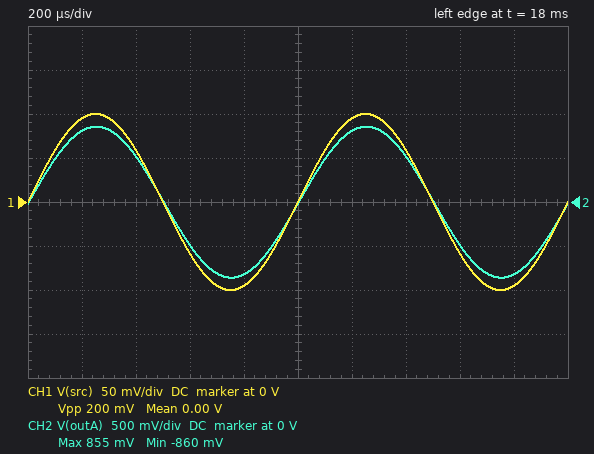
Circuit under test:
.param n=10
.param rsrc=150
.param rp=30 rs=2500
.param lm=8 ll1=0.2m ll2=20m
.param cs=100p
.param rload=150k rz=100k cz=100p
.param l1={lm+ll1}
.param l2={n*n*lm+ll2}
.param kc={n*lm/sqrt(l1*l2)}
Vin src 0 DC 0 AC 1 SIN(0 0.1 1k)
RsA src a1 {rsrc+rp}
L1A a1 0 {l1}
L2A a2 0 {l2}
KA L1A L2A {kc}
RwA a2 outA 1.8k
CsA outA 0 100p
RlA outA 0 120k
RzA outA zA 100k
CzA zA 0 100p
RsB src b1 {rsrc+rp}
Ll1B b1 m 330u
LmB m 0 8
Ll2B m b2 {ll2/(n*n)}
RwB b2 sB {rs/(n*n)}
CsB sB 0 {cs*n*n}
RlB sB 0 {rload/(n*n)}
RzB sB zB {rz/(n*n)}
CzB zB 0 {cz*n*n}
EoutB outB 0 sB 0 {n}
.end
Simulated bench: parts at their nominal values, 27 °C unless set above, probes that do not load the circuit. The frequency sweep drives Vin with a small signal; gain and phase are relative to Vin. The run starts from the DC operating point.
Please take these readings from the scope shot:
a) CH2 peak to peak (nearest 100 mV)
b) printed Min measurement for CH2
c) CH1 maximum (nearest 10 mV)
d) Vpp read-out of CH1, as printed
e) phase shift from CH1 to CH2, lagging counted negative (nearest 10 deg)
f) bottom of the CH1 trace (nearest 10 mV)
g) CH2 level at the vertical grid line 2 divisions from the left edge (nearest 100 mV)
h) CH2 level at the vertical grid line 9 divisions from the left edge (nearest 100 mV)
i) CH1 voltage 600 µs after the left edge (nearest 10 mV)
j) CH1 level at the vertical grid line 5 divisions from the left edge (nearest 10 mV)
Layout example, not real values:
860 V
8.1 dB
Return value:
1.7 V
-860 mV
100 mV
200 mV
0 deg
-100 mV
500 mV
-800 mV
-60 mV
0 V
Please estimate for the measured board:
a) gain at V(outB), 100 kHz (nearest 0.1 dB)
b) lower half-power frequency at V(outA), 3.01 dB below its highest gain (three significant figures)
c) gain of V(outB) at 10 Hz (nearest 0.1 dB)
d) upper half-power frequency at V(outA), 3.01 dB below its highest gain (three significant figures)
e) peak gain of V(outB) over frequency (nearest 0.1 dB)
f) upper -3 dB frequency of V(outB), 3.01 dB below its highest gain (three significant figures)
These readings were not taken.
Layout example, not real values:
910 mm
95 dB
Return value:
13.8 dB
3.12 Hz
18.5 dB
94.9 kHz
18.9 dB
84.9 kHz
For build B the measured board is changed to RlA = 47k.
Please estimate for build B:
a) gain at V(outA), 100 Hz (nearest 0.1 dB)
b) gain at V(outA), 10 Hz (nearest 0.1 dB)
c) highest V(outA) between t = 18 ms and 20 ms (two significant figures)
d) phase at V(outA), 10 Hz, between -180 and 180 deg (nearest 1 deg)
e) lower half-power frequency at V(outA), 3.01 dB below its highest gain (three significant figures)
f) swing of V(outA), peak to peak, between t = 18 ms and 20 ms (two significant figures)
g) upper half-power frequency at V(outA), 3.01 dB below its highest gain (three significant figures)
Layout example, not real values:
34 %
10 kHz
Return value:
16.9 dB
16.7 dB
700 mV
15 deg
2.62 Hz
1.4 V
97.7 kHz
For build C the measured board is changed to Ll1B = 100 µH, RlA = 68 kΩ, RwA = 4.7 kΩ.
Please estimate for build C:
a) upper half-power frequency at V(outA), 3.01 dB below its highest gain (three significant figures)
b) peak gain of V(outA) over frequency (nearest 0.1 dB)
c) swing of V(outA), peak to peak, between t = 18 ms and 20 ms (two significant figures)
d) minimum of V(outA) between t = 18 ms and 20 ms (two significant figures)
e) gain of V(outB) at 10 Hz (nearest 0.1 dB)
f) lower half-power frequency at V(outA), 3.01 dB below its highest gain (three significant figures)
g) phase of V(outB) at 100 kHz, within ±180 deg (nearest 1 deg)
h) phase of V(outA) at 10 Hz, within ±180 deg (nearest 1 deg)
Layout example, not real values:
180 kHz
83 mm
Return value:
89.8 kHz
17.5 dB
1.5 V
-750 mV
18.5 dB
2.87 Hz
-86 deg
16 deg
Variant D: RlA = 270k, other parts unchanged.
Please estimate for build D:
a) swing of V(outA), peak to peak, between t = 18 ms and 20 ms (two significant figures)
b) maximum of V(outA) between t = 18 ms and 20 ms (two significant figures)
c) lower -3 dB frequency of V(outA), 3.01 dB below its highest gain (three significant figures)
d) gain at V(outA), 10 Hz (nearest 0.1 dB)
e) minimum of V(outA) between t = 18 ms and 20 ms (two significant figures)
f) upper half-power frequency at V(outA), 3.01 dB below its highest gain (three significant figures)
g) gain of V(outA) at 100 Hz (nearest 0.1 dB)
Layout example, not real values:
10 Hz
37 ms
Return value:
1.9 V
930 mV
3.36 Hz
18.9 dB
-930 mV
93.4 kHz
19.4 dB
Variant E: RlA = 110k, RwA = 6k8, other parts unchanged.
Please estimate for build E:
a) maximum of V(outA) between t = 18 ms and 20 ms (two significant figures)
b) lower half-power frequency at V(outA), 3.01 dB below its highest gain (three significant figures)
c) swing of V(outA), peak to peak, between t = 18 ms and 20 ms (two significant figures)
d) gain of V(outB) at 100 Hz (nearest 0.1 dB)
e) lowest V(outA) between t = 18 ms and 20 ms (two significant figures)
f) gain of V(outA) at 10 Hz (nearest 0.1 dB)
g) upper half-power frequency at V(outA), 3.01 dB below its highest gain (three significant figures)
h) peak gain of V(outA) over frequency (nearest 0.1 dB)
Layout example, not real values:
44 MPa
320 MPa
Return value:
810 mV
3.10 Hz
1.6 V
18.9 dB
-820 mV
17.8 dB
80.9 kHz
18.2 dB
